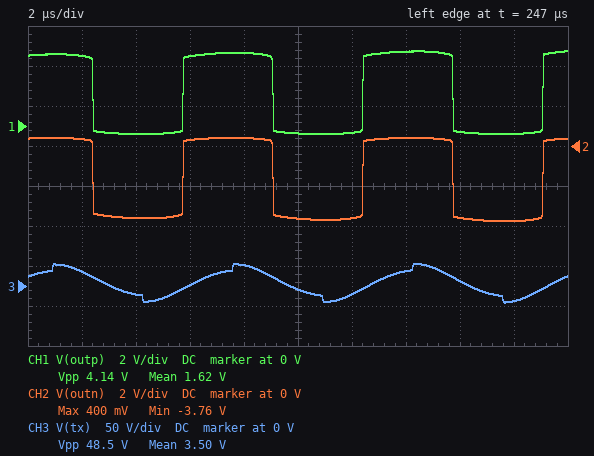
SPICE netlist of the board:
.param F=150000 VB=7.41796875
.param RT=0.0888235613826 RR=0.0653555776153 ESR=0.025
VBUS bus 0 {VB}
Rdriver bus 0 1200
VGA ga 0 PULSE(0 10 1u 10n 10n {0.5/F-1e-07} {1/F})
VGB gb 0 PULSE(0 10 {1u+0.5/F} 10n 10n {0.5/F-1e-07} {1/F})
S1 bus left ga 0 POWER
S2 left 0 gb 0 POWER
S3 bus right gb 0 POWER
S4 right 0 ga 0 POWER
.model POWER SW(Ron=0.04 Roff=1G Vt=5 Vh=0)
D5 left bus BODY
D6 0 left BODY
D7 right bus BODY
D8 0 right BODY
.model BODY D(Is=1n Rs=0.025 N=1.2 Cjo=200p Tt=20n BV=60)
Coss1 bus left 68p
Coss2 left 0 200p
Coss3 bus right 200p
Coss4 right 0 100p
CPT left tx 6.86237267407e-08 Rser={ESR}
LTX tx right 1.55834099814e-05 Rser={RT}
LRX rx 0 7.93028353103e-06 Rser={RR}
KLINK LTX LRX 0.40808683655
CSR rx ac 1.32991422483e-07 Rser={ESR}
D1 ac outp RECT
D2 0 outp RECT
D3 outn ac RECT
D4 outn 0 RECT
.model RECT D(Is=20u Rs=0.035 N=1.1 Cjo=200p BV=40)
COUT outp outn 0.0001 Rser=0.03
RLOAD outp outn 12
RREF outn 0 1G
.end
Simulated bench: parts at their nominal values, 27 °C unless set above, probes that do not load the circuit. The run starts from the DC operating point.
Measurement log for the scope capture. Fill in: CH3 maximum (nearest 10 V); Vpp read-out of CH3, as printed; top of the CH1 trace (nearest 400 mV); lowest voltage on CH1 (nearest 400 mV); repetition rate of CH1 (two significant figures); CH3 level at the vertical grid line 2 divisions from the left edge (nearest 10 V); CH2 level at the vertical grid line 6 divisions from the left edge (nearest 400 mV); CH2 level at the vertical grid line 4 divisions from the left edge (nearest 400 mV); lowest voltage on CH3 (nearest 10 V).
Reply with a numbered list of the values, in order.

1. 30 V
2. 48.5 V
3. 3.6 V
4. -400 mV
5. 150 kHz
6. -10 V
7. -3.6 V
8. 400 mV
9. -20 V
